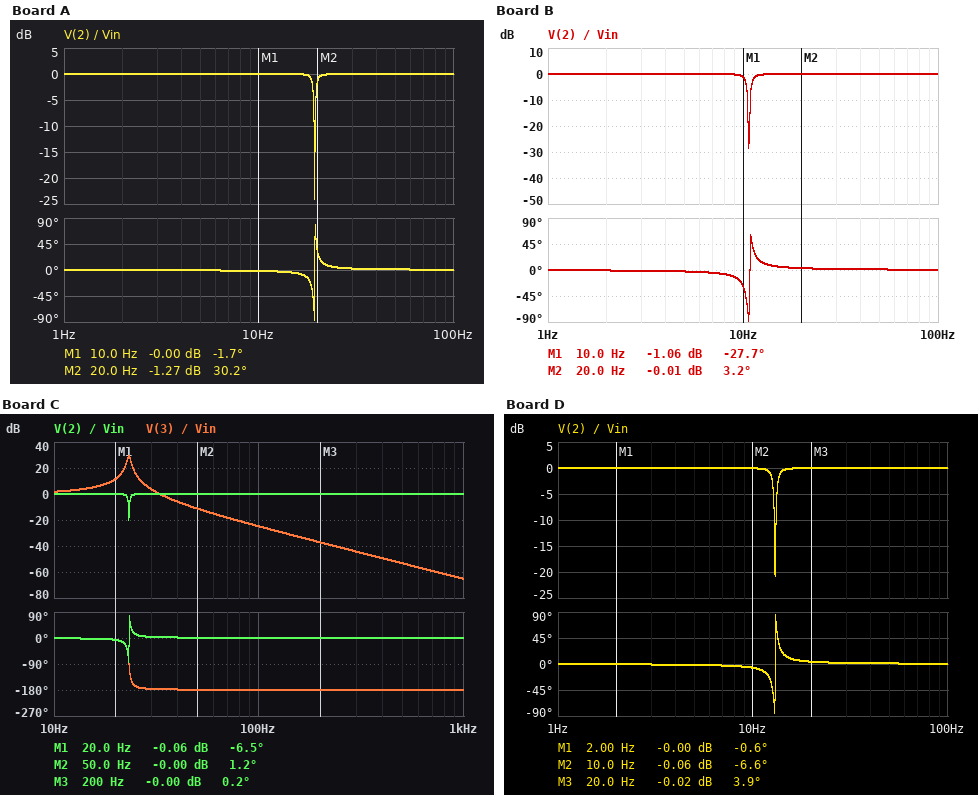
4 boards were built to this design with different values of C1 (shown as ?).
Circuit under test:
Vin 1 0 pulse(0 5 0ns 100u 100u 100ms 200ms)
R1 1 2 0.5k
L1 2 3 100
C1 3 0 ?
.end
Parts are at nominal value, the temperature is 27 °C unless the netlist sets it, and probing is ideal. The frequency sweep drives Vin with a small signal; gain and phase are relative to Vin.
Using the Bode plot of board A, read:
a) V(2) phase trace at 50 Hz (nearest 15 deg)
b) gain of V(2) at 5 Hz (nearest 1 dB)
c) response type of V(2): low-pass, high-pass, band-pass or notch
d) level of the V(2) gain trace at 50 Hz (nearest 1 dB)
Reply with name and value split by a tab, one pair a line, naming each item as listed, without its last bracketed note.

V(2) phase trace at 50 Hz	0 deg
gain of V(2) at 5 Hz	0 dB
response type of V(2): low-pass, high-pass, band-pass or notch	notch
level of the V(2) gain trace at 50 Hz	0 dB
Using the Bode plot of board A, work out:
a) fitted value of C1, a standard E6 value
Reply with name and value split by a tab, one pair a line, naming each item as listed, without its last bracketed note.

fitted value of C1, a standard E6 value	680 nF
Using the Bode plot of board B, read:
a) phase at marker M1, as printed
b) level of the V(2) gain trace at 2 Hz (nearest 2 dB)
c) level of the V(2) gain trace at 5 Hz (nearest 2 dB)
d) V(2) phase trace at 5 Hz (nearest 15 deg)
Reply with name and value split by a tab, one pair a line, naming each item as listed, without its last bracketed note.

phase at marker M1, as printed	-27.7 deg
level of the V(2) gain trace at 2 Hz	0 dB
level of the V(2) gain trace at 5 Hz	0 dB
V(2) phase trace at 5 Hz	0 deg
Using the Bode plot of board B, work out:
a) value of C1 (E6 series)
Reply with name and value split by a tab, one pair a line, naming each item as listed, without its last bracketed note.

value of C1	2.2 µF
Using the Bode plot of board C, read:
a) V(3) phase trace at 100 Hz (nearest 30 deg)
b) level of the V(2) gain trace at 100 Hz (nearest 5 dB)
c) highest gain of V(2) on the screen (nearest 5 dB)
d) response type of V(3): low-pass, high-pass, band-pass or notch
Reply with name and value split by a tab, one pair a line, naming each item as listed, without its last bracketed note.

V(3) phase trace at 100 Hz	-180 deg
level of the V(2) gain trace at 100 Hz	0 dB
highest gain of V(2) on the screen	0 dB
response type of V(3): low-pass, high-pass, band-pass or notch	band-pass
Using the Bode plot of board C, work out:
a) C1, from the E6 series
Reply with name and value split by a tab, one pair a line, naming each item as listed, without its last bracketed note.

C1, from the E6 series	470 nF
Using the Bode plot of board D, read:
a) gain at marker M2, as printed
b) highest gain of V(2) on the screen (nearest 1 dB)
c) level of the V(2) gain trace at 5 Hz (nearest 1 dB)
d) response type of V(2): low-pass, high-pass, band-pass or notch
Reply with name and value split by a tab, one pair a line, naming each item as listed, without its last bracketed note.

gain at marker M2, as printed	-0.06 dB
highest gain of V(2) on the screen	0 dB
level of the V(2) gain trace at 5 Hz	0 dB
response type of V(2): low-pass, high-pass, band-pass or notch	notch
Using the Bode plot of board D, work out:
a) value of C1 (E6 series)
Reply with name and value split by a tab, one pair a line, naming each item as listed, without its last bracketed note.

value of C1	1.5 µF
